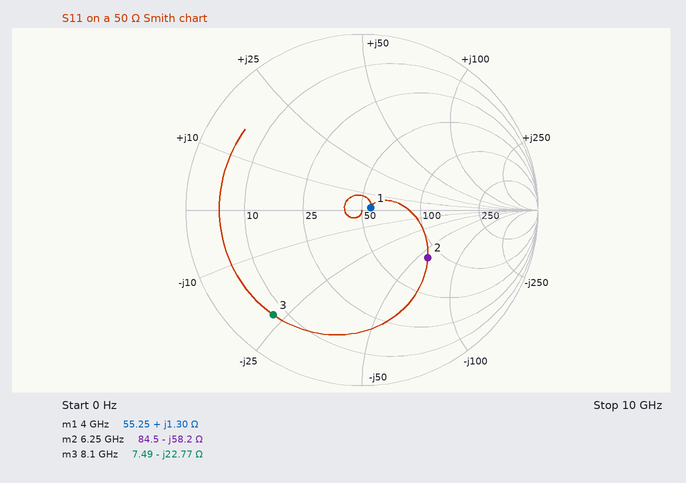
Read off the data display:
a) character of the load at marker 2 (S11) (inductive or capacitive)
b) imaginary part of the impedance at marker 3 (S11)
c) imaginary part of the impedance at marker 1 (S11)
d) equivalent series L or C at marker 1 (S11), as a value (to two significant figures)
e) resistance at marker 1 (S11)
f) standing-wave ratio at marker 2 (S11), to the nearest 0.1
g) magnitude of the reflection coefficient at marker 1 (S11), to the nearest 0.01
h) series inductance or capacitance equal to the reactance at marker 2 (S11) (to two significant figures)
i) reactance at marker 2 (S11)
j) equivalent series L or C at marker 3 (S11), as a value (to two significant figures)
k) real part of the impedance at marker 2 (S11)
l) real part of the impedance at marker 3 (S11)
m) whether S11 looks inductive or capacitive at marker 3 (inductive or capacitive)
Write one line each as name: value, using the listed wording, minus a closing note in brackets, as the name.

character of the load at marker 2 (S11): capacitive
imaginary part of the impedance at marker 3: -22.77 Ω
imaginary part of the impedance at marker 1: +1.30 Ω
equivalent series L or C at marker 1 (S11), as a value: 52 pH
resistance at marker 1: 55.25 Ω
standing-wave ratio at marker 2 (S11), to the nearest 0.1: 2.7
magnitude of the reflection coefficient at marker 1 (S11), to the nearest 0.01: 0.05
series inductance or capacitance equal to the reactance at marker 2 (S11): 440 fF
reactance at marker 2: -58.2 Ω
equivalent series L or C at marker 3 (S11), as a value: 860 fF
real part of the impedance at marker 2: 84.5 Ω
real part of the impedance at marker 3: 7.49 Ω
whether S11 looks inductive or capacitive at marker 3: capacitive
